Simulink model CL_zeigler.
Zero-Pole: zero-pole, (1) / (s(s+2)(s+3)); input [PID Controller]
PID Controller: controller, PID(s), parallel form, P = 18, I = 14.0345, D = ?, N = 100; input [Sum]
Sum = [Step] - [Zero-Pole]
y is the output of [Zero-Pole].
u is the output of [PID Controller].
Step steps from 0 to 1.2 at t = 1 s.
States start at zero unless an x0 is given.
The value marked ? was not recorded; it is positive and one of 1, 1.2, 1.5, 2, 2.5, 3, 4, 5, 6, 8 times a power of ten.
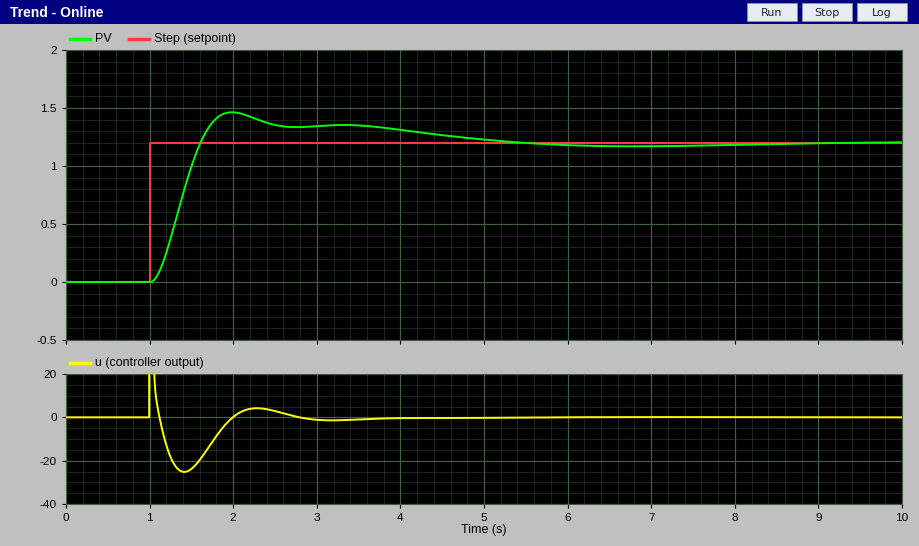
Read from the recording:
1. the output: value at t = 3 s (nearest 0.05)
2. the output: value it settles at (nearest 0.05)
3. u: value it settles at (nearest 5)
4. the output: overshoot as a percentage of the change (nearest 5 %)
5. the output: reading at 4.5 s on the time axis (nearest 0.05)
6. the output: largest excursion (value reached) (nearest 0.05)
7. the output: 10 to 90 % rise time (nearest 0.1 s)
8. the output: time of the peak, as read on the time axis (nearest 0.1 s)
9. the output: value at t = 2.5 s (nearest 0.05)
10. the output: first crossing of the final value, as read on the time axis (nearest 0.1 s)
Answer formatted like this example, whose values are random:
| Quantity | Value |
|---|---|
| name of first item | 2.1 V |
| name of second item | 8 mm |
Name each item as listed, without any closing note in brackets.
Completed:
| Quantity | Value |
|---|---|
| the output: value at t = 3 s | 1.35 |
| the output: value it settles at | 1.20 |
| u: value it settles at | 0 |
| the output: overshoot as a percentage of the change | 20 % |
| the output: reading at 4.5 s on the time axis | 1.25 |
| the output: largest excursion (value reached) | 1.45 |
| the output: 10 to 90 % rise time | 0.4 s |
| the output: time of the peak, as read on the time axis | 2.0 s |
| the output: value at t = 2.5 s | 1.35 |
| the output: first crossing of the final value, as read on the time axis | 1.6 s |
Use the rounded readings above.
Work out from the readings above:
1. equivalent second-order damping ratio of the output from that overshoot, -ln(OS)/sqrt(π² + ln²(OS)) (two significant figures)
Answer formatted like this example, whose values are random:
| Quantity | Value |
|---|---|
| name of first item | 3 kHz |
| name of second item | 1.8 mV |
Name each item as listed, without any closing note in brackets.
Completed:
| Quantity | Value |
|---|---|
| equivalent second-order damping ratio of the output from that overshoot, -ln(OS)/sqrt(π² + ln²(OS)) | 0.46 |
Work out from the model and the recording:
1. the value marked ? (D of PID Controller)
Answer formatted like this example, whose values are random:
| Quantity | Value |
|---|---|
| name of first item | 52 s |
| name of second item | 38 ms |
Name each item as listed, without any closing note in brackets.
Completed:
| Quantity | Value |
|---|---|
| the value marked ? | 15 |
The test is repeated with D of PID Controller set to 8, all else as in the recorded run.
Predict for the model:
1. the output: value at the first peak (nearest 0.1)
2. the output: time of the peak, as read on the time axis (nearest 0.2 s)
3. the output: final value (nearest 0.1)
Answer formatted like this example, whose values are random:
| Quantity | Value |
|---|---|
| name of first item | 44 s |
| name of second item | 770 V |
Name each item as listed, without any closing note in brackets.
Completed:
| Quantity | Value |
|---|---|
| the output: value at the first peak | 1.7 |
| the output: time of the peak, as read on the time axis | 2.4 s |
| the output: final value | 1.2 |
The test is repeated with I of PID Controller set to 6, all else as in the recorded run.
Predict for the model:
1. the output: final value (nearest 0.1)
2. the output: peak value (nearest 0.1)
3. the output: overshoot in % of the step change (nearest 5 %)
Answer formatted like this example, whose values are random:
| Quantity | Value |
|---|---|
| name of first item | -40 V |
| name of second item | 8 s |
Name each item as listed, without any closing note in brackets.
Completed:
| Quantity | Value |
|---|---|
| the output: final value | 1.2 |
| the output: peak value | 1.4 |
| the output: overshoot in % of the step change | 15 % |
